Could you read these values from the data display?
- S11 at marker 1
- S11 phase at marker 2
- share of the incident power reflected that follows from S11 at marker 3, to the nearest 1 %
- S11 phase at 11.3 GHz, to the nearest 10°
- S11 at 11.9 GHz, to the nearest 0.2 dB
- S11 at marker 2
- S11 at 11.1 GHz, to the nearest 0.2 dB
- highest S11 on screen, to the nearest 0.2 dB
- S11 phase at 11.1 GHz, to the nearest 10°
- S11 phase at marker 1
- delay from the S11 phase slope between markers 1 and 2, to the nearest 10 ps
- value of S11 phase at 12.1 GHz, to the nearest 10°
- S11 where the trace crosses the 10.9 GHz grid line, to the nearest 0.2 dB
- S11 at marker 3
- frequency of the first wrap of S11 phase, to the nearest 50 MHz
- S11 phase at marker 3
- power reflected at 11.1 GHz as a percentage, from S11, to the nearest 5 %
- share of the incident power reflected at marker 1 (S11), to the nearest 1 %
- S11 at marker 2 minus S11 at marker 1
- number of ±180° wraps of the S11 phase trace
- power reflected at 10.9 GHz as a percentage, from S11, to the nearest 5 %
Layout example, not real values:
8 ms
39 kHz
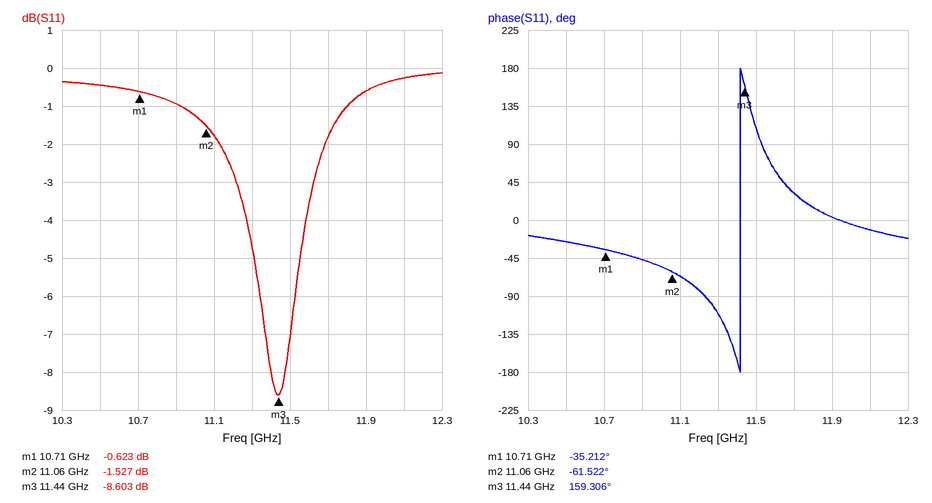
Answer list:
-0.623 dB
-61.522°
14 %
-110°
-0.6 dB
-1.527 dB
-1.8 dB
-0.2 dB
-70°
-35.212°
210 ps
-10°
-1.0 dB
-8.603 dB
11.40 GHz
159.306°
65 %
87 %
-0.904 dB
1
80 %
